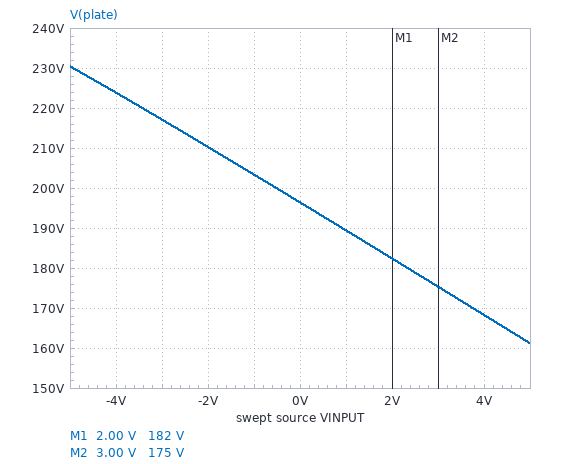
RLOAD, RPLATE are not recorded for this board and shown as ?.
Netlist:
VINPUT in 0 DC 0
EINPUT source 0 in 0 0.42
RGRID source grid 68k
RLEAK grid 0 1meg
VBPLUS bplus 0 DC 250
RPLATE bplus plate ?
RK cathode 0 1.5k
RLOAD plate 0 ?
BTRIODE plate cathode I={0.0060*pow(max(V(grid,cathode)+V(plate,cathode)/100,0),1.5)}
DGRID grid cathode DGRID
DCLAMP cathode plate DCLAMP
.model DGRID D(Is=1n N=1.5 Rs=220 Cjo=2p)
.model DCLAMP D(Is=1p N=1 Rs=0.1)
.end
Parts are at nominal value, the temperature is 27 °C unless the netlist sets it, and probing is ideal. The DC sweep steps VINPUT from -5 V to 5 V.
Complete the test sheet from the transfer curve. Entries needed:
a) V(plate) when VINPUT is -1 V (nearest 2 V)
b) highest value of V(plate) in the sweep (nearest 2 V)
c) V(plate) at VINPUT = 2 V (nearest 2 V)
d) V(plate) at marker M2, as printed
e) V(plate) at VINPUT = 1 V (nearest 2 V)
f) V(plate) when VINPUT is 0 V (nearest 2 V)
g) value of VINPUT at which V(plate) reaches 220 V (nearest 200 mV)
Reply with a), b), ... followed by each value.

a) 204 V
b) 230 V
c) 182 V
d) 175 V
e) 190 V
f) 196 V
g) -3.4 V
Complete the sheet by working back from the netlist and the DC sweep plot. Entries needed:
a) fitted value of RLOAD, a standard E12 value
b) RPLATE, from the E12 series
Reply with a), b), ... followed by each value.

a) 680 kΩ
b) 39 kΩ
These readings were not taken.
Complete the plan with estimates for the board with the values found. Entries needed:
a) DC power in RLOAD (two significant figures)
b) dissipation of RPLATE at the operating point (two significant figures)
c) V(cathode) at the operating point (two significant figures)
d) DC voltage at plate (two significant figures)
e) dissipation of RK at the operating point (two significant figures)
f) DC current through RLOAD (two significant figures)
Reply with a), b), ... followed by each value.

a) 57 mW
b) 74 mW
c) 1.6 V
d) 200 V
e) 1.8 mW
f) 290 µA
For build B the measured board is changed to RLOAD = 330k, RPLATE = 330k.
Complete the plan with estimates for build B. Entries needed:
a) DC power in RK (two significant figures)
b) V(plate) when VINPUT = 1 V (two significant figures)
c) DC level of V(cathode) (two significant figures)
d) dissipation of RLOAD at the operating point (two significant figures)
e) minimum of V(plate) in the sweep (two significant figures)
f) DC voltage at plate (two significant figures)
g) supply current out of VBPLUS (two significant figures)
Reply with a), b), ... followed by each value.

a) 180 µW
b) 49 V
c) 520 mV
d) 14 mW
e) 630 mV
f) 68 V
g) 550 µA
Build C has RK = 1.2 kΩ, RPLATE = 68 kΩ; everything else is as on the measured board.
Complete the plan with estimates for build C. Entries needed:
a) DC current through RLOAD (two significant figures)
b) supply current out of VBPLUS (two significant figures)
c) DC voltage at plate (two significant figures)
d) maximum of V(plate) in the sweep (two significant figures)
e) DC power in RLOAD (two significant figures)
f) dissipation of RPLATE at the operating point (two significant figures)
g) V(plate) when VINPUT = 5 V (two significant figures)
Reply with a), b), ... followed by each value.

a) 240 µA
b) 1.3 mA
c) 160 V
d) 220 V
e) 38 mW
f) 120 mW
g) 100 V
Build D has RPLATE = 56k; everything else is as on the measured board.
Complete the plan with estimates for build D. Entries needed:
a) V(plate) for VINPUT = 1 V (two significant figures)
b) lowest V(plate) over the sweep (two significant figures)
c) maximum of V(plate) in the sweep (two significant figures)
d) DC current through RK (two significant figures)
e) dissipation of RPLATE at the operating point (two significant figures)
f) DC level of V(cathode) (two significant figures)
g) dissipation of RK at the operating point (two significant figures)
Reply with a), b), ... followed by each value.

a) 170 V
b) 130 V
c) 220 V
d) 990 µA
e) 88 mW
f) 1.5 V
g) 1.5 mW
